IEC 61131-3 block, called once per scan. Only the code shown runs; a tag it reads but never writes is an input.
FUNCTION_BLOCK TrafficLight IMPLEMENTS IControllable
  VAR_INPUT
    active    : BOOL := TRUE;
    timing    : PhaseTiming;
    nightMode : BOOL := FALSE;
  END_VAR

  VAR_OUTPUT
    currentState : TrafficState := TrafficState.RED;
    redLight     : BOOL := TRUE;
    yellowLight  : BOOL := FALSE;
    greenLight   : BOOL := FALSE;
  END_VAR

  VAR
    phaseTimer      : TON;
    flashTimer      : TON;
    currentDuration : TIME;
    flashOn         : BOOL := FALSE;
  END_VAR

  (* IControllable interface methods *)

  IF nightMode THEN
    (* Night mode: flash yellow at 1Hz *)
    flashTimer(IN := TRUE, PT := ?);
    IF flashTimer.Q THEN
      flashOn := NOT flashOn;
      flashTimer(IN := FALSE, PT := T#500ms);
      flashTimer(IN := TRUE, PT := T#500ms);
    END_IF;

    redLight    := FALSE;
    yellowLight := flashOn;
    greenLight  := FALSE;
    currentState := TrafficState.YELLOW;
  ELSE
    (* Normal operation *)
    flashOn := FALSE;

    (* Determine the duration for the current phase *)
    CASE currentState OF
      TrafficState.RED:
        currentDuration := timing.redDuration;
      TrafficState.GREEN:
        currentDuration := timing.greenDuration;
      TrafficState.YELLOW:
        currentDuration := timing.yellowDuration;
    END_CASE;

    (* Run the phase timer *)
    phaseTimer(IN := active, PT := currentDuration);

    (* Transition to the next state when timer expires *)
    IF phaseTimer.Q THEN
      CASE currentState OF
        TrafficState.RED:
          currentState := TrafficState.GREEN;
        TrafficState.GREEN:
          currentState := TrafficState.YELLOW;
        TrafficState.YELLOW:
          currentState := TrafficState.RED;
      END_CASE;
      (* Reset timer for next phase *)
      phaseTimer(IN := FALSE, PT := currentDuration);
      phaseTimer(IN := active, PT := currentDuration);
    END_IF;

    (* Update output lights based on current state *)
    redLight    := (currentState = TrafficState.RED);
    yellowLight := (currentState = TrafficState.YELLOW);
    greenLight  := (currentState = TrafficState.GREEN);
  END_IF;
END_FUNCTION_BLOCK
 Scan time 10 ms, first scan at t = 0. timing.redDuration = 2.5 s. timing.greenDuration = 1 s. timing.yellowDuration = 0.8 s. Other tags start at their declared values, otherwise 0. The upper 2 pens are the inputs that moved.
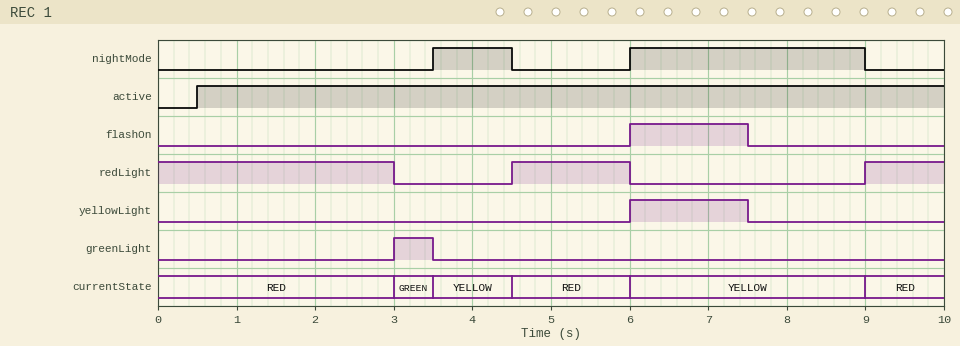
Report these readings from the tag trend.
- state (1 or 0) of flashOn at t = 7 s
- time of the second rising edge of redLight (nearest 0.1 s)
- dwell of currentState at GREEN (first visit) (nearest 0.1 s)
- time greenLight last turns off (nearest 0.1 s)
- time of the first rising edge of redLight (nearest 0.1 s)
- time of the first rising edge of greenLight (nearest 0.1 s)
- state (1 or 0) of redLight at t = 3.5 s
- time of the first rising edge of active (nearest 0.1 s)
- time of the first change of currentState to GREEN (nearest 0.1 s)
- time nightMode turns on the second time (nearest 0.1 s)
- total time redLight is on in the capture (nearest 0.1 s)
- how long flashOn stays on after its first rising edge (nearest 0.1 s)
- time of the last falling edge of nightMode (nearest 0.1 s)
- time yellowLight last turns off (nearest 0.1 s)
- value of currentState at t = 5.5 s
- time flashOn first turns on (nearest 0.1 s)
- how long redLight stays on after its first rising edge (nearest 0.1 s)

1
9.0 s
0.5 s
3.5 s
4.5 s
3.0 s
0
0.5 s
3.0 s
6.0 s
5.5 s
1.5 s
9.0 s
7.5 s
RED
6.0 s
1.5 s
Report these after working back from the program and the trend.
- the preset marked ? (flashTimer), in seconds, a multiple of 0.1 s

1.5 s
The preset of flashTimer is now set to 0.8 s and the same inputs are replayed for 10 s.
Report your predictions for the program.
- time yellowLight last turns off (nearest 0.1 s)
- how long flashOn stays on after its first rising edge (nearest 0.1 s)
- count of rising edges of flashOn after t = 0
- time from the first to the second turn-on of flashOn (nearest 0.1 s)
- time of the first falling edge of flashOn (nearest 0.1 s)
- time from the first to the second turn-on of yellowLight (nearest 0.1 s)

8.4 s
0.2 s
3
1.7 s
4.5 s
1.7 s
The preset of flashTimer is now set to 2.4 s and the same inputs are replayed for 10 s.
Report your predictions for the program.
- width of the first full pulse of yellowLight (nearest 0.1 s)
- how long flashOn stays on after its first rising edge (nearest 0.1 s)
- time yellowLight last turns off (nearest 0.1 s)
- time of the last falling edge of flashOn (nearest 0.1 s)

2.4 s
2.4 s
8.4 s
8.4 s
